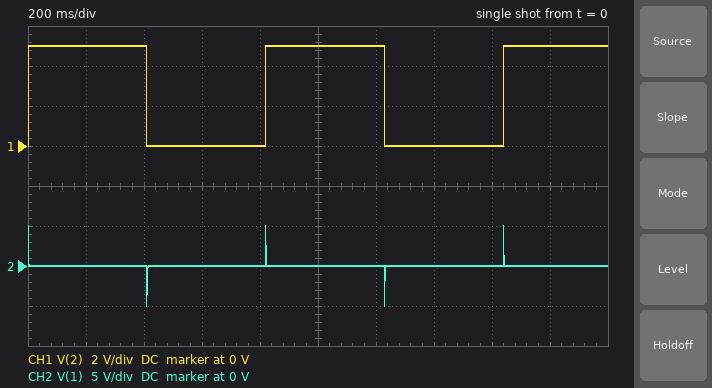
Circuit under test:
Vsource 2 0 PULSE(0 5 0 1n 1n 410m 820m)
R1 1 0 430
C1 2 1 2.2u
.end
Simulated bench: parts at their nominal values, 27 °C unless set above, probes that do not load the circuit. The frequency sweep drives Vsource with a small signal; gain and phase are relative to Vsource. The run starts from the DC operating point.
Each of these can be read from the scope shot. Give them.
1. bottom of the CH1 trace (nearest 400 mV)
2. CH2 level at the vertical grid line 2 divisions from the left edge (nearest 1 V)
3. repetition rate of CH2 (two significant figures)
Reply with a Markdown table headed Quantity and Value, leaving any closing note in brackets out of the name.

| Quantity | Value |
|---|---|
| bottom of the CH1 trace | 0 V |
| CH2 level at the vertical grid line 2 divisions from the left edge | 0 V |
| repetition rate of CH2 | 1.2 Hz |
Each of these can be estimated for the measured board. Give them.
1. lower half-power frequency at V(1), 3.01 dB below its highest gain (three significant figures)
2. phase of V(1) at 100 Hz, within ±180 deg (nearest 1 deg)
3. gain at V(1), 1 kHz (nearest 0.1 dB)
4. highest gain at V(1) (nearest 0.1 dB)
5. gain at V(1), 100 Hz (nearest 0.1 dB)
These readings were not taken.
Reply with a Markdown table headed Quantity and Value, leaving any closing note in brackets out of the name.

| Quantity | Value |
|---|---|
| lower half-power frequency at V(1), 3.01 dB below its highest gain | 168 Hz |
| phase of V(1) at 100 Hz, within ±180 deg | 59 deg |
| gain at V(1), 1 kHz | -0.1 dB |
| highest gain at V(1) | 0 dB |
| gain at V(1), 100 Hz | -5.8 dB |
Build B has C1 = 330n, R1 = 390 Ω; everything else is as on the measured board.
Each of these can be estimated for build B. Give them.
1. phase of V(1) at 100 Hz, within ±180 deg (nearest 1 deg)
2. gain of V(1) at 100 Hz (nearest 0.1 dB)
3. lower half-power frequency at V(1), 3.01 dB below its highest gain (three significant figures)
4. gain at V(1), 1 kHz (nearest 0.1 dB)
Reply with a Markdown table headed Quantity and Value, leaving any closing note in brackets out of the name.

| Quantity | Value |
|---|---|
| phase of V(1) at 100 Hz, within ±180 deg | 85 deg |
| gain of V(1) at 100 Hz | -21.9 dB |
| lower half-power frequency at V(1), 3.01 dB below its highest gain | 1.24 kHz |
| gain at V(1), 1 kHz | -4.0 dB |
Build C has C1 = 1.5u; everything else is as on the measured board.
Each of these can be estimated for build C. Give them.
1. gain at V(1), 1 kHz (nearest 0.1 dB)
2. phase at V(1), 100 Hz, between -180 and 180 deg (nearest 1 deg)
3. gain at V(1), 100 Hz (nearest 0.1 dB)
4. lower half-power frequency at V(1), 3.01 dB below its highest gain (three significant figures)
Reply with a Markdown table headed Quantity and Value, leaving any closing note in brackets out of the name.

| Quantity | Value |
|---|---|
| gain at V(1), 1 kHz | -0.3 dB |
| phase at V(1), 100 Hz, between -180 and 180 deg | 68 deg |
| gain at V(1), 100 Hz | -8.5 dB |
| lower half-power frequency at V(1), 3.01 dB below its highest gain | 247 Hz |
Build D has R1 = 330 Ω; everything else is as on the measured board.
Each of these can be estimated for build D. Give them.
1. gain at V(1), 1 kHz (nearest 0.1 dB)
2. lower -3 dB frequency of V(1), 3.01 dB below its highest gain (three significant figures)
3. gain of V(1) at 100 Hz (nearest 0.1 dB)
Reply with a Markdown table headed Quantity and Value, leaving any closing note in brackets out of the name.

| Quantity | Value |
|---|---|
| gain at V(1), 1 kHz | -0.2 dB |
| lower -3 dB frequency of V(1), 3.01 dB below its highest gain | 219 Hz |
| gain of V(1) at 100 Hz | -7.6 dB |
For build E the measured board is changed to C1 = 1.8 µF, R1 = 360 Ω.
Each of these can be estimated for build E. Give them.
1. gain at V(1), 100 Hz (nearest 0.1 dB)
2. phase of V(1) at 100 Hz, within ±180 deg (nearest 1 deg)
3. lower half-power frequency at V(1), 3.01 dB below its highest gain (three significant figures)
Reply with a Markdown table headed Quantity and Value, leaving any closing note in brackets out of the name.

| Quantity | Value |
|---|---|
| gain at V(1), 100 Hz | -8.5 dB |
| phase of V(1) at 100 Hz, within ±180 deg | 68 deg |
| lower half-power frequency at V(1), 3.01 dB below its highest gain | 246 Hz |
